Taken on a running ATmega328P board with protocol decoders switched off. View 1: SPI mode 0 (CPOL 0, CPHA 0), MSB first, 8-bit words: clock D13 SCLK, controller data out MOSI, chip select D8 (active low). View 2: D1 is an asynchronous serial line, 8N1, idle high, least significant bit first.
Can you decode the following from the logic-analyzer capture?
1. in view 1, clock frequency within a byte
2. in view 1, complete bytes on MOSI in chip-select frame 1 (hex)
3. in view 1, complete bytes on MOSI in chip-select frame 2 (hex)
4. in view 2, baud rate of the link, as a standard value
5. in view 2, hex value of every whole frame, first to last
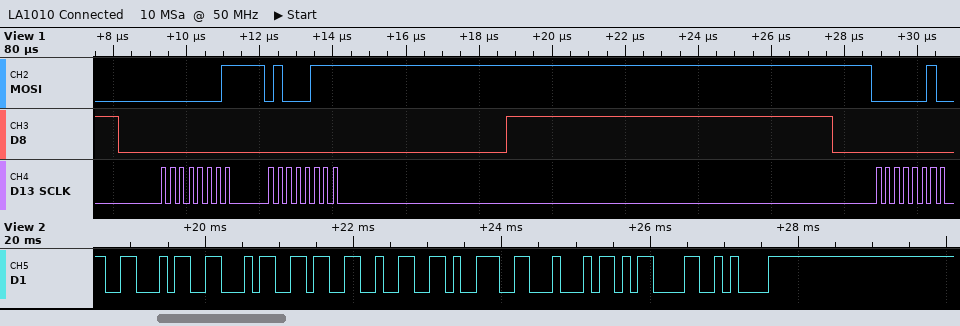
4 MHz
01 47
02
9600 baud
46 46 36 32 39 44 0D 0A
